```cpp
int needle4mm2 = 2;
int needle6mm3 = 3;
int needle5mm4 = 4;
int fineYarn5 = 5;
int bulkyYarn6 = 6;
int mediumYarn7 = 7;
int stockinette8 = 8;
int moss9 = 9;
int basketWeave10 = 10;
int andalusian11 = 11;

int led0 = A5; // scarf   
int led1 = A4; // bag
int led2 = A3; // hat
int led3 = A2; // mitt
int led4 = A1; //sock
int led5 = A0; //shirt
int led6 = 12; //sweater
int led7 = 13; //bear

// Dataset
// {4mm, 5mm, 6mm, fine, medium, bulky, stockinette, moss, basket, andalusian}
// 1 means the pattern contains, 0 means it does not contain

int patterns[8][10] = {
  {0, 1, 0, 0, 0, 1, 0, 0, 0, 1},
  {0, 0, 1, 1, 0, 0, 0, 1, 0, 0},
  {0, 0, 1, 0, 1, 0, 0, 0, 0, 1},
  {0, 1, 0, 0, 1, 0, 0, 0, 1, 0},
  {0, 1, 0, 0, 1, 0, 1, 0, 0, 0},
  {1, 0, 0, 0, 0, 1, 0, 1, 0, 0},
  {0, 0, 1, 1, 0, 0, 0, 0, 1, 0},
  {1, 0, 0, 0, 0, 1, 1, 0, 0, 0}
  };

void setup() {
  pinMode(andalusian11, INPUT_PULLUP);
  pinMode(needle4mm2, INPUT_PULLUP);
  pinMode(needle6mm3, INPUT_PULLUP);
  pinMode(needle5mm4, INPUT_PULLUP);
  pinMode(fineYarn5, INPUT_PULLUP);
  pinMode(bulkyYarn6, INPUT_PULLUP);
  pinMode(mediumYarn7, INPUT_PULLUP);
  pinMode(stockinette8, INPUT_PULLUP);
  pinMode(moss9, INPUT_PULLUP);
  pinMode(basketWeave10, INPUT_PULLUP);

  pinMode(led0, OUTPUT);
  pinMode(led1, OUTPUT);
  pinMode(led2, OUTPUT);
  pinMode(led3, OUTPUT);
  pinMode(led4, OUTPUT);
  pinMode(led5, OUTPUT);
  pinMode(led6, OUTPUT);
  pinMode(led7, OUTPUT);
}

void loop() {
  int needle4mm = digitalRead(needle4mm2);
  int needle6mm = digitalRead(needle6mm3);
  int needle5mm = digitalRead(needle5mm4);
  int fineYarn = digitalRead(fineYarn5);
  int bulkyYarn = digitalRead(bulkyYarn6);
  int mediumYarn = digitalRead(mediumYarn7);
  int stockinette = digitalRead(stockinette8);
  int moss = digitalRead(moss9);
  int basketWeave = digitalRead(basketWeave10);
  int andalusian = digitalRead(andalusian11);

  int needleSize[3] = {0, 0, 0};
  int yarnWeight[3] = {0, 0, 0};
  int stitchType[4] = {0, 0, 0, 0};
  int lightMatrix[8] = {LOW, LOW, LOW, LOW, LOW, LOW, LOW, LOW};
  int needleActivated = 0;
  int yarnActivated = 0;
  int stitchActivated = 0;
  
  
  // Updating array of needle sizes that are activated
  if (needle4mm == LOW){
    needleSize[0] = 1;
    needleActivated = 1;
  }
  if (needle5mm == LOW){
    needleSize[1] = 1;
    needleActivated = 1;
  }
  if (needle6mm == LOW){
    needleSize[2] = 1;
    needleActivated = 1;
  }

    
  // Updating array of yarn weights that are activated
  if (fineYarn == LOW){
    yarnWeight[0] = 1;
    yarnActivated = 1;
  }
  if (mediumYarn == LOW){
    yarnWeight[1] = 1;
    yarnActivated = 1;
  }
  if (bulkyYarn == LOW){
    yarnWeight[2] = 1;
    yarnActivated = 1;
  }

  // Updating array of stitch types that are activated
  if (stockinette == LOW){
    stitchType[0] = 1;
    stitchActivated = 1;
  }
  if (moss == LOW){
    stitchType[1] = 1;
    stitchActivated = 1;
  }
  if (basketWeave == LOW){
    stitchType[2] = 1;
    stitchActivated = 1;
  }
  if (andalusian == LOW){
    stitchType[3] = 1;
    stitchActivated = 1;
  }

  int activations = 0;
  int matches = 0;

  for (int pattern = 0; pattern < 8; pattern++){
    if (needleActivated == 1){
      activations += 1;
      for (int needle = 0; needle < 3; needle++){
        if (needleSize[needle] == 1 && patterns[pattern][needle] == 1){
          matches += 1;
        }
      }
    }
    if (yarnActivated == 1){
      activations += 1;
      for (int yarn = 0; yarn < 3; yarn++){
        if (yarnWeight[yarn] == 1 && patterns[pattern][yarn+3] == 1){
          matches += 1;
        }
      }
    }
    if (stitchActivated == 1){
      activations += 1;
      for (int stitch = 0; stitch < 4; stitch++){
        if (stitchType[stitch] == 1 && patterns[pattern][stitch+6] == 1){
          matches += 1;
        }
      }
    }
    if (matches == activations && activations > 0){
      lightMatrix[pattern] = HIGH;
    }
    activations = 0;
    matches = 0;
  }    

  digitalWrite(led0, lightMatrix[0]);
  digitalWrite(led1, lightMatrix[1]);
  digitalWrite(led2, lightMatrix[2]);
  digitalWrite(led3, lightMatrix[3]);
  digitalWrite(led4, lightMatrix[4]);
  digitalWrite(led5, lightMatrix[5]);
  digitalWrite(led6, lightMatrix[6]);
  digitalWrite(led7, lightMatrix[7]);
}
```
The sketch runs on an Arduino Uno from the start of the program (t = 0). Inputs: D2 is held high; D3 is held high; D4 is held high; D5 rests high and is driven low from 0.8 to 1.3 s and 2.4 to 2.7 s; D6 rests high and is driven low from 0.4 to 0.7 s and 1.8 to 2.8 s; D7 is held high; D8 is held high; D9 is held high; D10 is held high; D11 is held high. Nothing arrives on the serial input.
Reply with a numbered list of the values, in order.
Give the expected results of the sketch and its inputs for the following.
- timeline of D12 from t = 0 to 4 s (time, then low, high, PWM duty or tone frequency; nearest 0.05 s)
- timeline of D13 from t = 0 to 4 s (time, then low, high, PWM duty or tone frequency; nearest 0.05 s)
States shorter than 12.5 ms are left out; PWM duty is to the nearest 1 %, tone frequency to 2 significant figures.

1. 0 s low; 0.8 s high; 1.3 s low; 2.4 s high; 2.7 s low
2. 0 s low; 0.4 s high; 0.7 s low; 1.8 s high; 2.8 s low
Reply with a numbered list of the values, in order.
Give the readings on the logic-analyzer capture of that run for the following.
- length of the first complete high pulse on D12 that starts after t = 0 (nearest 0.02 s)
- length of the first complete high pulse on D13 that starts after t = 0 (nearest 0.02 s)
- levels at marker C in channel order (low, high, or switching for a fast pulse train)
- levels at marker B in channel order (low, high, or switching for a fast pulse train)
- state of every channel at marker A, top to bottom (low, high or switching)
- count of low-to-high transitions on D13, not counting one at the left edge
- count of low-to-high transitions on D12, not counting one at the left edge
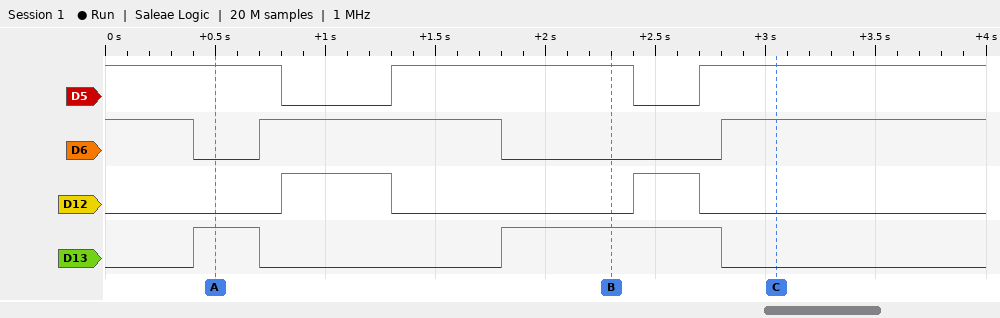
1. 0.50 s
2. 0.30 s
3. D5 high, D6 high, D12 low, D13 low
4. D5 high, D6 low, D12 low, D13 high
5. D5 high, D6 low, D12 low, D13 high
6. 2
7. 2
